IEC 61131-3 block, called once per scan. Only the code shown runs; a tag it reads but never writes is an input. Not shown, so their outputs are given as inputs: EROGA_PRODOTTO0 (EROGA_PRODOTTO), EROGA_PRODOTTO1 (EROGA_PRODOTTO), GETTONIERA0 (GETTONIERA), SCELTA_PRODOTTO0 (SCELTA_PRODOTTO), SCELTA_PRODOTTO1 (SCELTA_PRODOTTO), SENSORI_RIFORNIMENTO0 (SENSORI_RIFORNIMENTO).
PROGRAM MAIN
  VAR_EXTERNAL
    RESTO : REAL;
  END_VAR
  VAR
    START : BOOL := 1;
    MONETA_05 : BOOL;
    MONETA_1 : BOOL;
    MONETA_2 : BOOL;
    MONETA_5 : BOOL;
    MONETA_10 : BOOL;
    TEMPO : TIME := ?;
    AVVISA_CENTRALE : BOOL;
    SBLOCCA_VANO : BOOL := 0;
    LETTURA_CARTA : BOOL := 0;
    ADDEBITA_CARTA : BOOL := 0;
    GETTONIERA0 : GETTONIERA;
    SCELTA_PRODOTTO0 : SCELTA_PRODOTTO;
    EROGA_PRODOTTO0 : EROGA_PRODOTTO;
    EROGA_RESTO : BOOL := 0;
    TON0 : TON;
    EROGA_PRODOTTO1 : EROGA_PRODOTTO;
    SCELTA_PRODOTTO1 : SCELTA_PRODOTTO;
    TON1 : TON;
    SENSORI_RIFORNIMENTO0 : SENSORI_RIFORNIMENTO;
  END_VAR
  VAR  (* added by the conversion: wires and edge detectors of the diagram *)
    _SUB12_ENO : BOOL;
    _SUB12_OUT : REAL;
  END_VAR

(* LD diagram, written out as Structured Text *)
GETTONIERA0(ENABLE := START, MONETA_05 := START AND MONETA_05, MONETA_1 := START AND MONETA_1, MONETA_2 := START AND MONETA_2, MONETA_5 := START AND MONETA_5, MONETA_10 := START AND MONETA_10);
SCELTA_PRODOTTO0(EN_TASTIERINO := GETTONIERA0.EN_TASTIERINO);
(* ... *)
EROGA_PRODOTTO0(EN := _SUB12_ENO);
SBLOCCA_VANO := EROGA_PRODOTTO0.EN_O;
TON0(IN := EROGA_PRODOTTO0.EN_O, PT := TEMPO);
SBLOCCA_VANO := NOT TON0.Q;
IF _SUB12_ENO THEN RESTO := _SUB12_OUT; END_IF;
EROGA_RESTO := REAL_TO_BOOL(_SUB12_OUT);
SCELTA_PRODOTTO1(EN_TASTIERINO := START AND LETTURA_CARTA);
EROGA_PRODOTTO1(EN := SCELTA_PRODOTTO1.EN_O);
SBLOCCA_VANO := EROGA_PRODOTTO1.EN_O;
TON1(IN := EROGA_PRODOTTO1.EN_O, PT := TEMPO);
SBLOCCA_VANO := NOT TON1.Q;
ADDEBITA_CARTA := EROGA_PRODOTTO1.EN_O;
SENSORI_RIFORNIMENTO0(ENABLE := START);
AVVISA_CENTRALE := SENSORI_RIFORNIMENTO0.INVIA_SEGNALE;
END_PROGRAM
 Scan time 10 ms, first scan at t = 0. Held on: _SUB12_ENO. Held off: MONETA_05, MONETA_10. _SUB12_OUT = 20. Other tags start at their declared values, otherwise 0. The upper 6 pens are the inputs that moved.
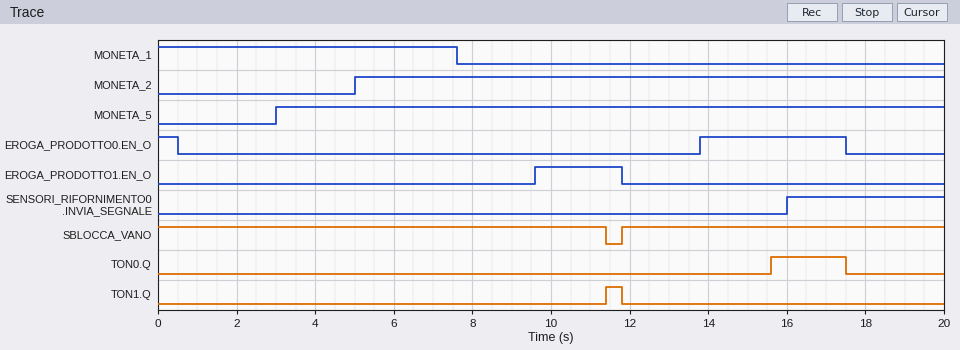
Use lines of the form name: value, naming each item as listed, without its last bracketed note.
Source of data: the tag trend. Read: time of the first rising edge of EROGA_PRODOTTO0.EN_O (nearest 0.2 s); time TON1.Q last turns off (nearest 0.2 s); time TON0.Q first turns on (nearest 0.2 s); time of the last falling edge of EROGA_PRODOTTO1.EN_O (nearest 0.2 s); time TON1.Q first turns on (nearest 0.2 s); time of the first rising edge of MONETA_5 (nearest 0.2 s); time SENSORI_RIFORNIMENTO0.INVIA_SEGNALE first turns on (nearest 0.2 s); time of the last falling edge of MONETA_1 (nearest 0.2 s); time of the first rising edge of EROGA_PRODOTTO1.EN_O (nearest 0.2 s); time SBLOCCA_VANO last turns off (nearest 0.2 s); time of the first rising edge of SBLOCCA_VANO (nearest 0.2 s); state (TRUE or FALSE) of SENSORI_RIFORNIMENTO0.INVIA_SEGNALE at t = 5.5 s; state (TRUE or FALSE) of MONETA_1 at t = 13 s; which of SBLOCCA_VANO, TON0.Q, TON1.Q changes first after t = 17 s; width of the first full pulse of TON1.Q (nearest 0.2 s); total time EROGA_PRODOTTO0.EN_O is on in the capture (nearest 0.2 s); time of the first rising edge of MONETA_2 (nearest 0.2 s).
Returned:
time of the first rising edge of EROGA_PRODOTTO0.EN_O: 13.8 s
time TON1.Q last turns off: 11.8 s
time TON0.Q first turns on: 15.6 s
time of the last falling edge of EROGA_PRODOTTO1.EN_O: 11.8 s
time TON1.Q first turns on: 11.4 s
time of the first rising edge of MONETA_5: 3.0 s
time SENSORI_RIFORNIMENTO0.INVIA_SEGNALE first turns on: 16.0 s
time of the last falling edge of MONETA_1: 7.6 s
time of the first rising edge of EROGA_PRODOTTO1.EN_O: 9.6 s
time SBLOCCA_VANO last turns off: 11.4 s
time of the first rising edge of SBLOCCA_VANO: 11.8 s
state (TRUE or FALSE) of SENSORI_RIFORNIMENTO0.INVIA_SEGNALE at t = 5.5 s: FALSE
state (TRUE or FALSE) of MONETA_1 at t = 13 s: FALSE
which of SBLOCCA_VANO, TON0.Q, TON1.Q changes first after t = 17 s: TON0.Q
width of the first full pulse of TON1.Q: 0.4 s
total time EROGA_PRODOTTO0.EN_O is on in the capture: 4.2 s
time of the first rising edge of MONETA_2: 5.0 s
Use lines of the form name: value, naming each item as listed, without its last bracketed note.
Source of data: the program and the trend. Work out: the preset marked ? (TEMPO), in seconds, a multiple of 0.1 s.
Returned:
the preset marked ? (TEMPO), in seconds, a multiple of 0.1 s: 1.8 s
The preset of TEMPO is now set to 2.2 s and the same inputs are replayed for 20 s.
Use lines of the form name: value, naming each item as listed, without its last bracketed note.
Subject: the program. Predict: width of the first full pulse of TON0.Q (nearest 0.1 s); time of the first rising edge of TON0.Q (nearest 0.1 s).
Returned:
width of the first full pulse of TON0.Q: 1.5 s
time of the first rising edge of TON0.Q: 16.0 s
